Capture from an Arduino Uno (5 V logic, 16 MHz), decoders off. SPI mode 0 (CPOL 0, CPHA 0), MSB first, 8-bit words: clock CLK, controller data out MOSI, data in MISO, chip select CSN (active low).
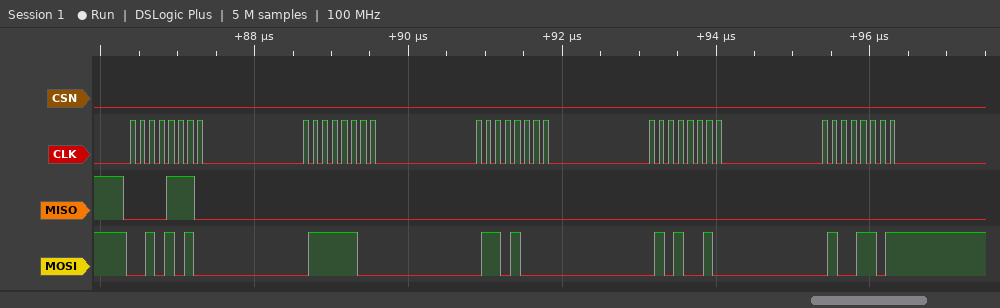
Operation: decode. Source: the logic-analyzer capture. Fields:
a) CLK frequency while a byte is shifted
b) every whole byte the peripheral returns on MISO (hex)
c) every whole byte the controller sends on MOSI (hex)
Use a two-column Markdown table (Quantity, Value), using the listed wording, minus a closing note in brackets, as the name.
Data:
| Quantity | Value |
|---|---|
| CLK frequency while a byte is shifted | 8 MHz |
| every whole byte the peripheral returns on MISO | 0E 00 00 00 00 |
| every whole byte the controller sends on MOSI | 2A 7C 68 52 4D |
